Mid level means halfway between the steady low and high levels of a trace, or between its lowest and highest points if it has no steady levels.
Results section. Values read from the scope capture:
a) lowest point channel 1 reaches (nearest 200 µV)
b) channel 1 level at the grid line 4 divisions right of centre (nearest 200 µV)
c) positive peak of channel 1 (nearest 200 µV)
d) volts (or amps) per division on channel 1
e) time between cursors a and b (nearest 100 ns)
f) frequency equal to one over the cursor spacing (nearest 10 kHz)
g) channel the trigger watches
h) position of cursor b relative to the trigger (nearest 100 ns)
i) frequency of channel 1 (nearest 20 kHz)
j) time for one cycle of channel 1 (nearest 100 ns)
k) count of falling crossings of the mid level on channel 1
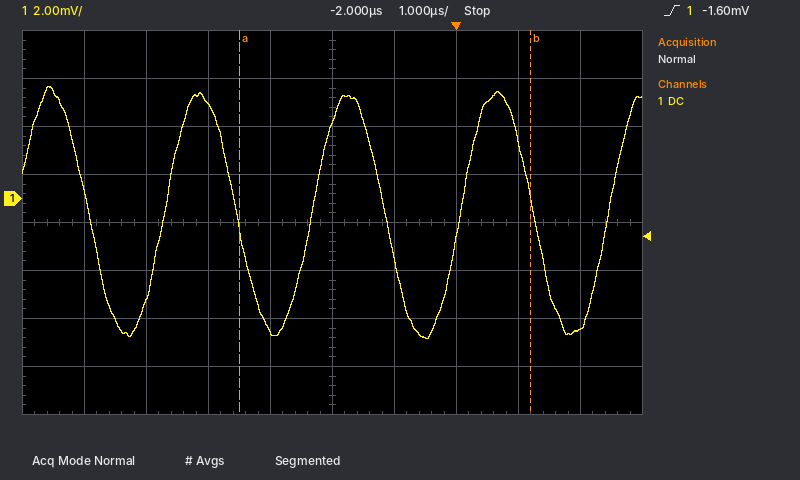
-5.8 mV
-5.4 mV
4.6 mV
2 mV
4.7 µs
210 kHz
channel 1
+1.2 µs
420 kHz
2.4 µs
4
